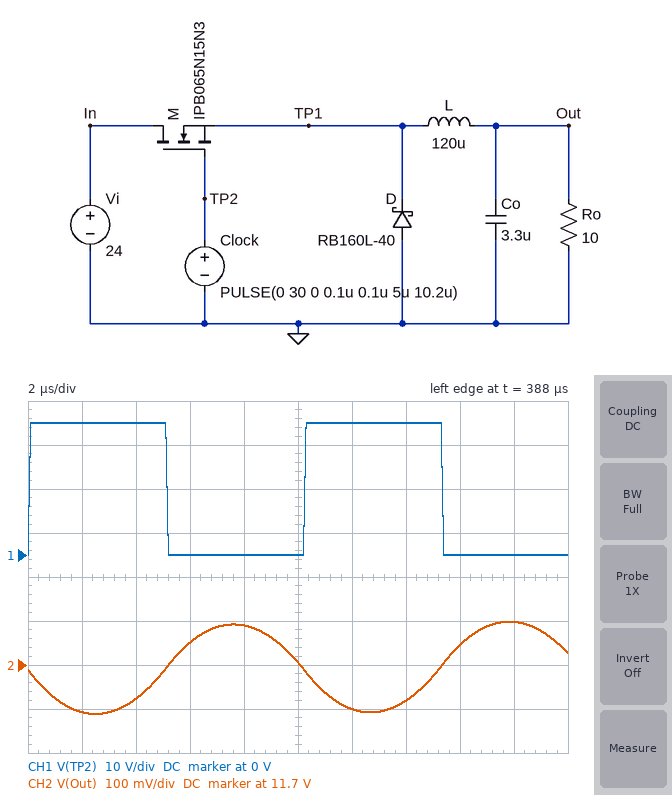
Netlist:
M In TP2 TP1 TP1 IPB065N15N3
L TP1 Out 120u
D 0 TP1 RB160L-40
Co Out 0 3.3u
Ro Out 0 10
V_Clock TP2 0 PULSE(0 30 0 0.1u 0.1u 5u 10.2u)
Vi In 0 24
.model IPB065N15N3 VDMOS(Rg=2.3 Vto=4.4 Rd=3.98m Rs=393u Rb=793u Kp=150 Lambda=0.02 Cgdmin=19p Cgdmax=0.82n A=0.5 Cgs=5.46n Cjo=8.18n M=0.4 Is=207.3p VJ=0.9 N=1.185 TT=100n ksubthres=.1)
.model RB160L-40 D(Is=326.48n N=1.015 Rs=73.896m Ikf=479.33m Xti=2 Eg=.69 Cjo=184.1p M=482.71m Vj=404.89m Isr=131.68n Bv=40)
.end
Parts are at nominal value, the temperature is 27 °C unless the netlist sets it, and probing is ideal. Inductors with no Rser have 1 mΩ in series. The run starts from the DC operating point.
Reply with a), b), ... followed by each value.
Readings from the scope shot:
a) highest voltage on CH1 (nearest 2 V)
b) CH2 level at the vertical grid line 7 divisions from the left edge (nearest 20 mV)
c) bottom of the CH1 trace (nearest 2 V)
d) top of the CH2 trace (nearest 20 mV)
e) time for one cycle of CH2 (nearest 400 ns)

a) 30 V
b) 11.62 V
c) 0 V
d) 11.80 V
e) 10.0 µs
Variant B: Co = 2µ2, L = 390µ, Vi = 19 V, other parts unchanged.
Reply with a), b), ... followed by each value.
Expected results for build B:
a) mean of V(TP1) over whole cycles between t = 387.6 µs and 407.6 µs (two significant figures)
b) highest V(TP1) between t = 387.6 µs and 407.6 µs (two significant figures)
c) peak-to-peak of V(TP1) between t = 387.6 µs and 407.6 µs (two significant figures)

a) 9.3 V
b) 19 V
c) 20 V
